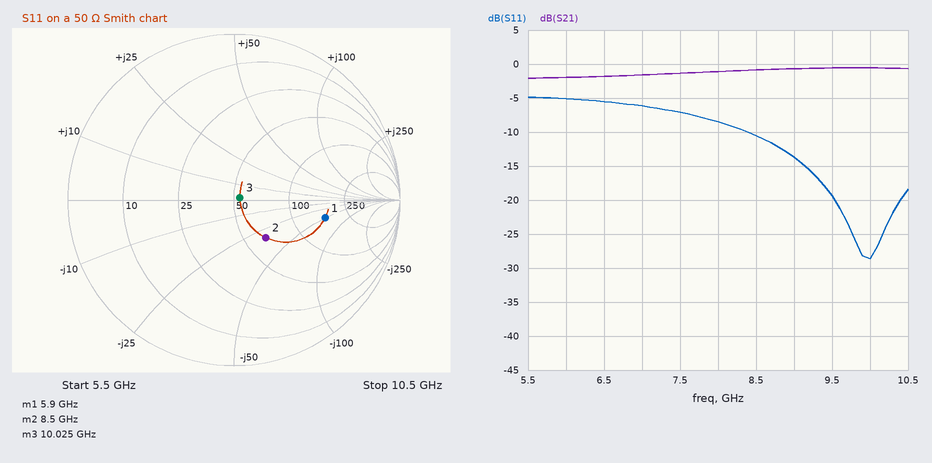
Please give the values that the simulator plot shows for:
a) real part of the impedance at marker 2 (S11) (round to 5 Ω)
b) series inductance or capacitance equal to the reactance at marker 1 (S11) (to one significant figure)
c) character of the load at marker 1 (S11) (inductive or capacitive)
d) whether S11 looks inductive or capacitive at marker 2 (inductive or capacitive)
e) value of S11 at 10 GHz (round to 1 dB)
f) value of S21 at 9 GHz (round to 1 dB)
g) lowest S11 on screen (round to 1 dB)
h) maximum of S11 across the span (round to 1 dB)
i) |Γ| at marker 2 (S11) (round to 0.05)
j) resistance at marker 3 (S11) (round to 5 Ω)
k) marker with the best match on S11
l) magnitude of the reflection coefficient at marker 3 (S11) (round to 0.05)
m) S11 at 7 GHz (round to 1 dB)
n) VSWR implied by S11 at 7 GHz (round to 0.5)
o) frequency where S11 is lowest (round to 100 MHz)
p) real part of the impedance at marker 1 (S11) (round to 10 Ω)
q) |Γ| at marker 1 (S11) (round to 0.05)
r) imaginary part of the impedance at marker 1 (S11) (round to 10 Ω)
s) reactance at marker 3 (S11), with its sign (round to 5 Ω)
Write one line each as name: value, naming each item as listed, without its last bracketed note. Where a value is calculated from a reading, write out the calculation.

real part of the impedance at marker 2 (S11): 65 Ω
series inductance or capacitance equal to the reactance at marker 1 (S11): C = 1/(2π × 5.9 GHz × 50 Ω) ≈ 540 fF, so 500 fF to one significant figure
character of the load at marker 1 (S11): capacitive
whether S11 looks inductive or capacitive at marker 2: capacitive
value of S11 at 10 GHz: -29 dB
value of S21 at 9 GHz: -1 dB
lowest S11 on screen: -29 dB
maximum of S11 across the span: -5 dB
|Γ| at marker 2 (S11): 0.30
resistance at marker 3 (S11): 55 Ω
marker with the best match on S11: marker 3
magnitude of the reflection coefficient at marker 3 (S11): 0.05
S11 at 7 GHz: -6 dB
VSWR implied by S11 at 7 GHz: |Γ| = 10^(-6/20) = 0.5012; VSWR = (1 + 0.5012)/(1 − 0.5012) ≈ 3.0
frequency where S11 is lowest: 10.0 GHz
real part of the impedance at marker 1 (S11): 160 Ω
|Γ| at marker 1 (S11): 0.55
imaginary part of the impedance at marker 1 (S11): -50 Ω
reactance at marker 3 (S11), with its sign: 0 Ω
